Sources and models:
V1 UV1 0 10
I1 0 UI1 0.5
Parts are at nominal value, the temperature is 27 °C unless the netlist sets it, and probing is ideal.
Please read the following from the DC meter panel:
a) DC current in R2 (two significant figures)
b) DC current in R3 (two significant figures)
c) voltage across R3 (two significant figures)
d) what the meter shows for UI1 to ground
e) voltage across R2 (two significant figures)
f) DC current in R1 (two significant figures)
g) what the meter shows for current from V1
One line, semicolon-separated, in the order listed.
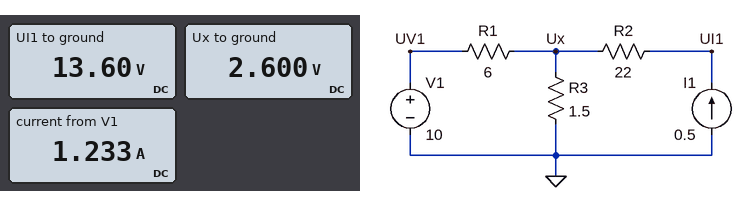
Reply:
500 mA; 1.7 A; 2.6 V; 13.60 V; 11 V; 1.2 A; 1.233 A
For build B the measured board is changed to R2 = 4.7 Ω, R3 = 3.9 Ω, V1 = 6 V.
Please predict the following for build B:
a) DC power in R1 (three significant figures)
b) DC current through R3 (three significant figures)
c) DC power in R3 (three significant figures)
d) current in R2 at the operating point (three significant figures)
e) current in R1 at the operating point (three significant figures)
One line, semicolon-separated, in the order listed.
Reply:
1.00 W; 909 mA; 3.22 W; 500 mA; 409 mA
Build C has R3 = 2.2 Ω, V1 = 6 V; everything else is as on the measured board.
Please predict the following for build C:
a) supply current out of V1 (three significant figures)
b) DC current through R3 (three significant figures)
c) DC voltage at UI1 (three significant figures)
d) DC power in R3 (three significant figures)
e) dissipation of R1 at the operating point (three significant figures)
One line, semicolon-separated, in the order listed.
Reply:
598 mA; 1.10 A; 13.4 V; 2.65 W; 2.14 W
